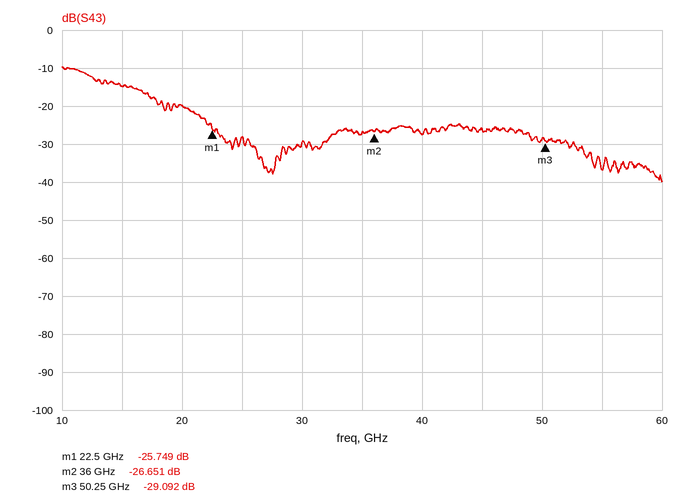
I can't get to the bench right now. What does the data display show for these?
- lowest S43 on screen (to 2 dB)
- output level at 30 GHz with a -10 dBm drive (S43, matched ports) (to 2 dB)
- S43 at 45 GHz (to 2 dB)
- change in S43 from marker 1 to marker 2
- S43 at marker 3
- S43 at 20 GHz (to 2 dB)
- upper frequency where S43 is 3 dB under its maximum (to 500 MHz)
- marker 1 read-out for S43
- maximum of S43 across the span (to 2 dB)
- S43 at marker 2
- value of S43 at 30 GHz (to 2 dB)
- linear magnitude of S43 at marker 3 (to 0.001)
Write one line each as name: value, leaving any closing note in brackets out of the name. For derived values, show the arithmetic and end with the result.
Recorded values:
lowest S43 on screen: -40 dB
output level at 30 GHz with a -10 dBm drive (S43, matched ports): -10 dBm + (-30 dB) = -40 dBm
S43 at 45 GHz: -26 dB
change in S43 from marker 1 to marker 2: -26.651 − (-25.749) = -0.902 dB
S43 at marker 3: -29.092 dB
S43 at 20 GHz: -20 dB
upper frequency where S43 is 3 dB under its maximum: 12.5 GHz
marker 1 read-out for S43: -25.749 dB
maximum of S43 across the span: -10 dB
S43 at marker 2: -26.651 dB
value of S43 at 30 GHz: -30 dB
linear magnitude of S43 at marker 3: 10^(-29.092/20) ≈ 0.035
